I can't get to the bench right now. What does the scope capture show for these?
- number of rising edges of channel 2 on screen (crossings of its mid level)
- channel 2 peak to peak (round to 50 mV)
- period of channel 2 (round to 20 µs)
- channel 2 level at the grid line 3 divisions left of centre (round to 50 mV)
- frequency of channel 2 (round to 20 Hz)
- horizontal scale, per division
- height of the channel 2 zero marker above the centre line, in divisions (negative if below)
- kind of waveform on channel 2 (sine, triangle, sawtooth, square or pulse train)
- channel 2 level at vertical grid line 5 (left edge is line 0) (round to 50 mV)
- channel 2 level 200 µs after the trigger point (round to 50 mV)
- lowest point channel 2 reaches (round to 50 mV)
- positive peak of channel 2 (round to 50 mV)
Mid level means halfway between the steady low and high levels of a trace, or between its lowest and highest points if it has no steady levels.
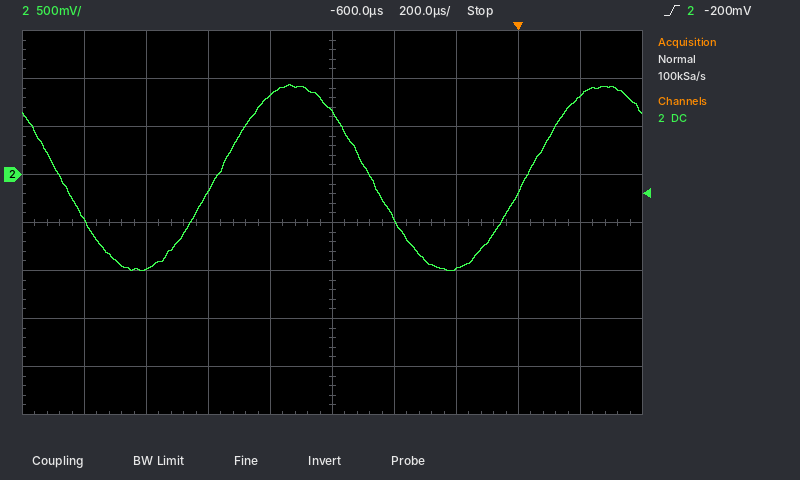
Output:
2
1.95 V
1.00 ms
-1.00 V
1.00 kHz
200 µs
+1.0 div
sine
650 mV
800 mV
-1.00 V
950 mV
